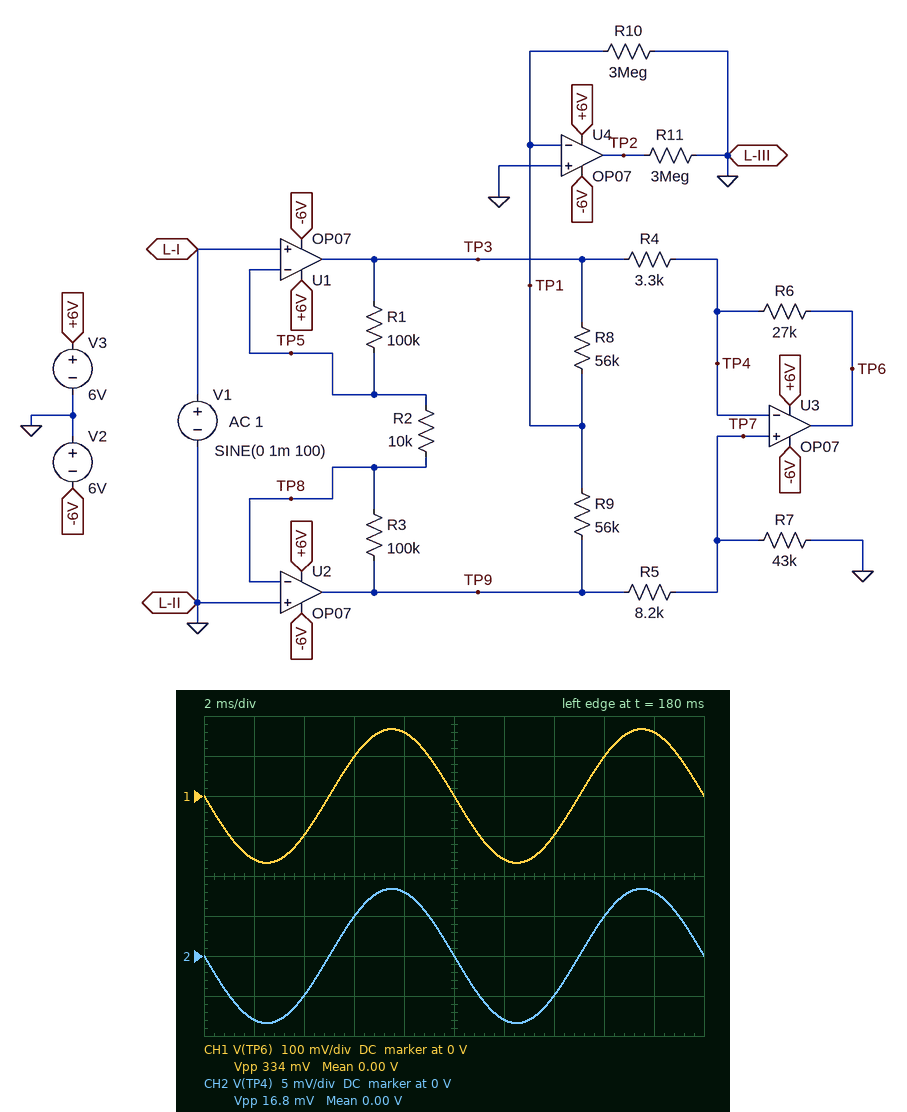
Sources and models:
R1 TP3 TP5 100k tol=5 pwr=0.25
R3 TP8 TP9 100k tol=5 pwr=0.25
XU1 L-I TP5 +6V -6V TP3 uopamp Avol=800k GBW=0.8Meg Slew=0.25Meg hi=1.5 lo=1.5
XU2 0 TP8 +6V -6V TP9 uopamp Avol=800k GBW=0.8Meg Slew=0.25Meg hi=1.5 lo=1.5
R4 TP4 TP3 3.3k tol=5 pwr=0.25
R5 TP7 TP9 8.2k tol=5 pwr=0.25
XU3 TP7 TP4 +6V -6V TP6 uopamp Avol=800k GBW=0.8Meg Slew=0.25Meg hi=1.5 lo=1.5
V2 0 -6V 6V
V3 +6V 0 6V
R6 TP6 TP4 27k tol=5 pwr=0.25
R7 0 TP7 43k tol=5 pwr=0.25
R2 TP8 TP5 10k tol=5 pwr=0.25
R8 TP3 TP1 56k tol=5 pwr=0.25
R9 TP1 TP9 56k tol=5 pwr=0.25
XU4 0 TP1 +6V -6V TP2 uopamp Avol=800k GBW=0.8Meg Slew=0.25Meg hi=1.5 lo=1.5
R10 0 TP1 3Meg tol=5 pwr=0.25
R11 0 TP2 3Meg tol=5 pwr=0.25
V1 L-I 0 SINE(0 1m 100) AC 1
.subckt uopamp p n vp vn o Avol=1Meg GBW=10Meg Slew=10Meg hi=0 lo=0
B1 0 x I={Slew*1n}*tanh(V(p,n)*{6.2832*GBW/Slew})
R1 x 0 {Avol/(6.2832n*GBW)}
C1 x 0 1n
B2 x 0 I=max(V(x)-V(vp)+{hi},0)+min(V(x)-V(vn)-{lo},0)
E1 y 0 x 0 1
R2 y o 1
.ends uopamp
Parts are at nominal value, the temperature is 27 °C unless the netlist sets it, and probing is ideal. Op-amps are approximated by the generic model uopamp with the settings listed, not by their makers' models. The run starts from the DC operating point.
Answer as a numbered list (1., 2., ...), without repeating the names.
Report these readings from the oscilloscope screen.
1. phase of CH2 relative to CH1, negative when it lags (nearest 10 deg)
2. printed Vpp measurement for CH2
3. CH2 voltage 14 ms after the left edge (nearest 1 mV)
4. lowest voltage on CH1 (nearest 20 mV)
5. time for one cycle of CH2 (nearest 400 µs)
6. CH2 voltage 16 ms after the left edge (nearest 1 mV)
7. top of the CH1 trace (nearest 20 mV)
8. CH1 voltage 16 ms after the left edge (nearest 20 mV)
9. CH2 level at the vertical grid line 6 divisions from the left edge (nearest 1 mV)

1. 0 deg
2. 16.8 mV
3. -5 mV
4. -160 mV
5. 10.0 ms
6. 5 mV
7. 160 mV
8. 100 mV
9. -8 mV
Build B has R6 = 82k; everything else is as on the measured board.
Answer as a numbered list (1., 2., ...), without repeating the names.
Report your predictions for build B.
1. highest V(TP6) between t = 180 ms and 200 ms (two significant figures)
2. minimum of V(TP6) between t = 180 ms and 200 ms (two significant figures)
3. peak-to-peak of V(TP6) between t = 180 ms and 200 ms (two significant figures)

1. 490 mV
2. -490 mV
3. 980 mV
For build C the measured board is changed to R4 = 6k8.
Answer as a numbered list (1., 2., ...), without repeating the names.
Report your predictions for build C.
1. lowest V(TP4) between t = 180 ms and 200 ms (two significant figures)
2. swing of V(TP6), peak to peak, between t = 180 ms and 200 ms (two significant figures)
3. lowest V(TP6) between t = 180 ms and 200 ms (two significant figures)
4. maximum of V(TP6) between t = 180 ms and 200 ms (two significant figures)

1. -8.4 mV
2. 170 mV
3. -85 mV
4. 85 mV
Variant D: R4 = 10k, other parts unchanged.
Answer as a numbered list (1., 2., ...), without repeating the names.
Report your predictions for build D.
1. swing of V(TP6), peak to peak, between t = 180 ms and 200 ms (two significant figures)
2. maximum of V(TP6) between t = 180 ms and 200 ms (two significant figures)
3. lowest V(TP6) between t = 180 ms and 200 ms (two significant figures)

1. 120 mV
2. 61 mV
3. -61 mV
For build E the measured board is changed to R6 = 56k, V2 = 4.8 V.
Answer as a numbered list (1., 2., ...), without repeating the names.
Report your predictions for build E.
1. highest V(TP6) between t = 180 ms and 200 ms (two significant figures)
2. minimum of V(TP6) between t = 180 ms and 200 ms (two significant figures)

1. 340 mV
2. -340 mV
